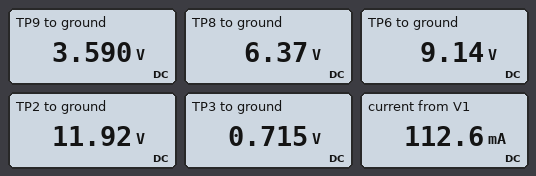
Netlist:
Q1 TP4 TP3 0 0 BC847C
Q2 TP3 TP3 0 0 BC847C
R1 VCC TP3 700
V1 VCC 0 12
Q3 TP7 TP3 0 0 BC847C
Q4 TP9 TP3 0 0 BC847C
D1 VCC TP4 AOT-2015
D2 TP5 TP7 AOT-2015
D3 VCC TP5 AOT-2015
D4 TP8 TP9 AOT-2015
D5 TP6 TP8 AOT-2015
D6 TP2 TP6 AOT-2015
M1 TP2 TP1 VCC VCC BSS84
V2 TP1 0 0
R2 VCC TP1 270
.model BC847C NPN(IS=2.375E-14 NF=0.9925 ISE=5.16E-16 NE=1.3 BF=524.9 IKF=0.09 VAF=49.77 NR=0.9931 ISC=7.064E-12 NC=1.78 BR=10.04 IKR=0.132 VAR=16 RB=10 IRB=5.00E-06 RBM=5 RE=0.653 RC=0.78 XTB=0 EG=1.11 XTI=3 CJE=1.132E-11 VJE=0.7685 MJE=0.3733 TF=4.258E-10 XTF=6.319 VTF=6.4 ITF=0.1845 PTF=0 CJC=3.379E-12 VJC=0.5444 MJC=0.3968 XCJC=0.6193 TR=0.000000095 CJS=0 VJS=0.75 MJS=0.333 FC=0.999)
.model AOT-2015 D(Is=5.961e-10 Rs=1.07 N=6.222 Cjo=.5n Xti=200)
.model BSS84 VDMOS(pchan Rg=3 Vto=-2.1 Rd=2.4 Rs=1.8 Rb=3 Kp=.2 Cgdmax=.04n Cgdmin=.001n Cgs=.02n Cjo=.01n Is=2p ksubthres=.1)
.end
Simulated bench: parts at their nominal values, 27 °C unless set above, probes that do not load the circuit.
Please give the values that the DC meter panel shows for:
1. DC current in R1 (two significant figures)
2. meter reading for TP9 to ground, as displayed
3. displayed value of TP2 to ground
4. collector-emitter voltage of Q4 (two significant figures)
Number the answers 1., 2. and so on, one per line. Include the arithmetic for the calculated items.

1. (12 V - 715 mV) / 700 Ω = 16 mA
2. 3.590 V
3. 11.92 V
4. 3.59 V = 3.6 V
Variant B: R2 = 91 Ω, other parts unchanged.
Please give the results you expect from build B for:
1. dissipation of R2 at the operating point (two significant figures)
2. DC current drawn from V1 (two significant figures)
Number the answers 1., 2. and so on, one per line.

1. 1.6 W
2. 200 mA
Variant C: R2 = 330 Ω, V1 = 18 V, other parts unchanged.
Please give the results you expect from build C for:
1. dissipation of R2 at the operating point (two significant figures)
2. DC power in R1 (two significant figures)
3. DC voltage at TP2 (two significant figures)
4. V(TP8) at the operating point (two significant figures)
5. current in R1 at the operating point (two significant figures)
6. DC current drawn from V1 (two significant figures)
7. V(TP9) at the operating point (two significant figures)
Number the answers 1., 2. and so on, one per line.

1. 980 mW
2. 430 mW
3. 18 V
4. 12 V
5. 25 mA
6. 160 mA
7. 9.3 V
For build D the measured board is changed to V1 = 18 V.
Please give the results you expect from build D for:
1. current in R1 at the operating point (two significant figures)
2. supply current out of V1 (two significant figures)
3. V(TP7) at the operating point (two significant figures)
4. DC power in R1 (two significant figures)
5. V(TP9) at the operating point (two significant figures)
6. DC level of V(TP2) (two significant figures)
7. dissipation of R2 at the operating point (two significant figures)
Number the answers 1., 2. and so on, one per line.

1. 25 mA
2. 180 mA
3. 12 V
4. 430 mW
5. 9.3 V
6. 18 V
7. 1.2 W
